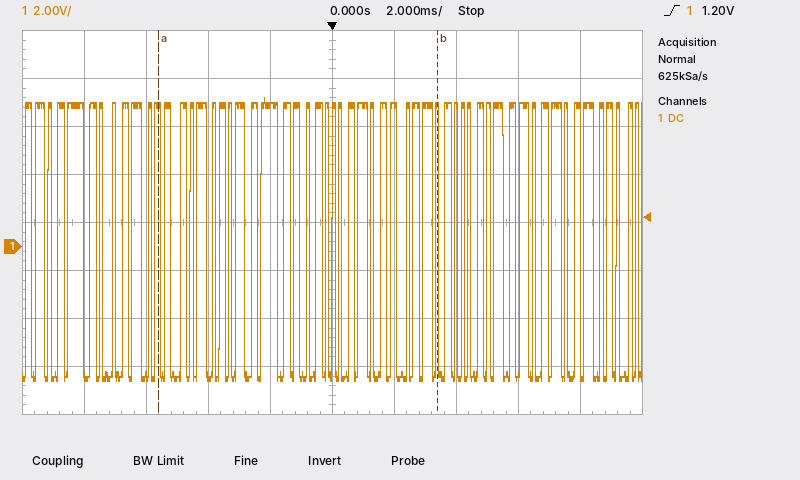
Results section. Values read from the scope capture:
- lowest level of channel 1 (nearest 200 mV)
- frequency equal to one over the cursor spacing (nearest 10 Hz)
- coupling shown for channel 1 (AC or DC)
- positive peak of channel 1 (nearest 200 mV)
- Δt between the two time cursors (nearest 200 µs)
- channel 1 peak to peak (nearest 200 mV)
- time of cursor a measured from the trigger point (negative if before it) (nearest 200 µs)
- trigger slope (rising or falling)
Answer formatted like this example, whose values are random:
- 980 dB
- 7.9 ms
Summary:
- -5.6 V
- 110 Hz
- DC
- 6.2 V
- 9.0 ms
- 11.8 V
- -5.6 ms
- rising
